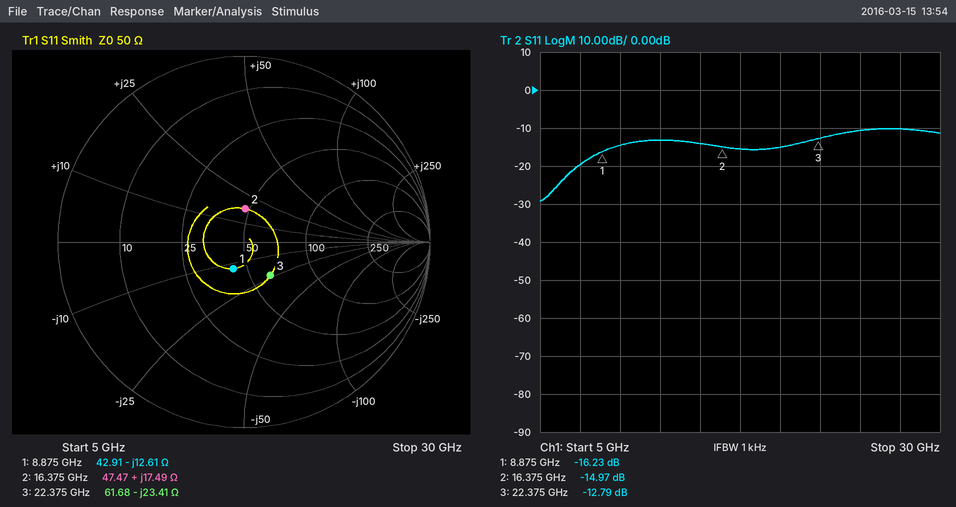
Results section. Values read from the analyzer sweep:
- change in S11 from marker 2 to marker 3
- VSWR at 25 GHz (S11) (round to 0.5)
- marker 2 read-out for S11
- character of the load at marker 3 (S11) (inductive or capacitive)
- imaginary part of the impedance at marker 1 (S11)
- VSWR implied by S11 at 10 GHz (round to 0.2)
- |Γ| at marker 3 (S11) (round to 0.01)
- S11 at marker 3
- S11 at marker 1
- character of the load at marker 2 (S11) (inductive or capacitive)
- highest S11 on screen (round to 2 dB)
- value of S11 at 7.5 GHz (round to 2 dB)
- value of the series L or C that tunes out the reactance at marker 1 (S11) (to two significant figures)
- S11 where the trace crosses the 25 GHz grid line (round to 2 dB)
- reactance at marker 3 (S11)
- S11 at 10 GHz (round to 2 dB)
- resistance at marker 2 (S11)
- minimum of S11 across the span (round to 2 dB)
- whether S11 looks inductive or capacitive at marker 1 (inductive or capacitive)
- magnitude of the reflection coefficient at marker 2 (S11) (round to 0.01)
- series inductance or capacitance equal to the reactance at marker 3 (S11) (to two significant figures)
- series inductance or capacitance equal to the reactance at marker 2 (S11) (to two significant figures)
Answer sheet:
2.18 dB
2.0
-14.97 dB
capacitive
-12.61 Ω
1.4
0.23
-12.79 dB
-16.23 dB
inductive
-10 dB
-20 dB
230 pH
-10 dB
-23.41 Ω
-14 dB
47.47 Ω
-30 dB
capacitive
0.18
300 fF
170 pH
